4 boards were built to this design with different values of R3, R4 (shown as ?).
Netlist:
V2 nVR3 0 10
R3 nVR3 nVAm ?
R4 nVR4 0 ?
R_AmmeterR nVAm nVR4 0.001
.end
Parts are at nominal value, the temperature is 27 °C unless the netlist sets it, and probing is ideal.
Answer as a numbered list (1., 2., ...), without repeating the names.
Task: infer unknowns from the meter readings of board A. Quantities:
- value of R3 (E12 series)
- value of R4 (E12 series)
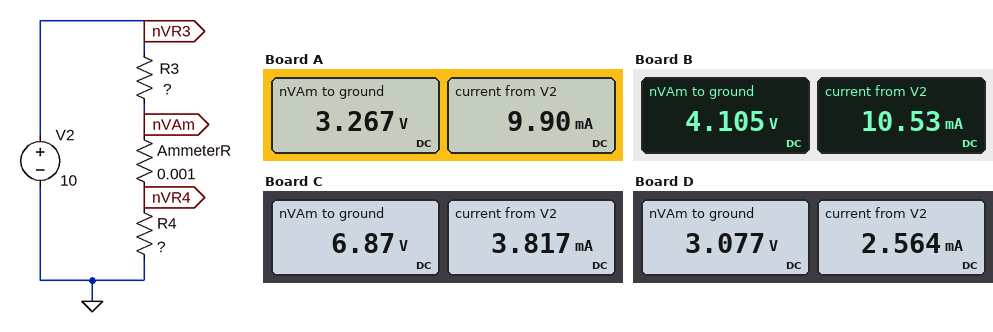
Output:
1. 680 Ω
2. 330 Ω
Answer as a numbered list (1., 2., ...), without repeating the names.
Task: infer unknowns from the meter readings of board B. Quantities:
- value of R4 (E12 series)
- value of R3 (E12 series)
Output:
1. 390 Ω
2. 560 Ω
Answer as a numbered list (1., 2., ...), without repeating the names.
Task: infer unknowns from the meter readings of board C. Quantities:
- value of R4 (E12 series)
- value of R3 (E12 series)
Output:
1. 1.8 kΩ
2. 820 Ω
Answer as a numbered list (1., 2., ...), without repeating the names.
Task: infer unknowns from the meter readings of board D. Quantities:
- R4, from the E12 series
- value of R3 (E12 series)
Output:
1. 1.2 kΩ
2. 2.7 kΩ
